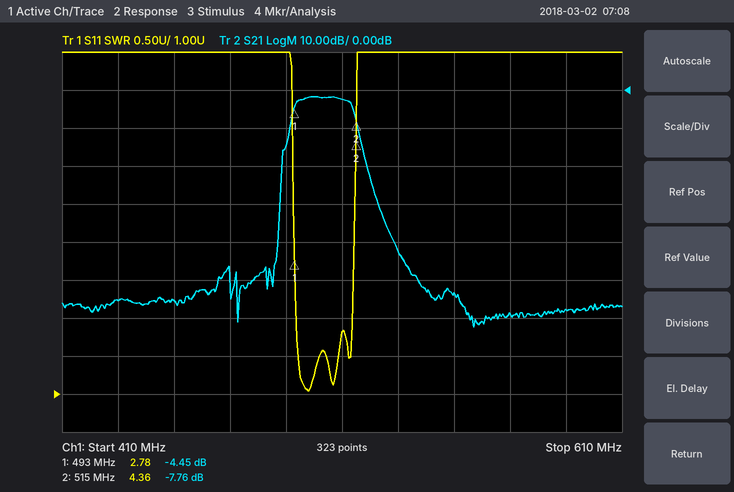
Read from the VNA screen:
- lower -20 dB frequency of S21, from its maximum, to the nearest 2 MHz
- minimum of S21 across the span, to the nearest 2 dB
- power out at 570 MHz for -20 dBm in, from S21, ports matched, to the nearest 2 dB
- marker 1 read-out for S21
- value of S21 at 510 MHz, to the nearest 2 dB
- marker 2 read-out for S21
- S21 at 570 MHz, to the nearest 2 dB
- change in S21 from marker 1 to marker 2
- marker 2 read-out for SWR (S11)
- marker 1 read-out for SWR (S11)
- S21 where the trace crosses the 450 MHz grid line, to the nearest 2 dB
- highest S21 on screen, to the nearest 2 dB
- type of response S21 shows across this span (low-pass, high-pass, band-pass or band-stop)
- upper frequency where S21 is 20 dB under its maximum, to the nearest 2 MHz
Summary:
488 MHz
-62 dB
-78 dBm
-4.45 dB
-2 dB
-7.76 dB
-58 dB
-3.31 dB
4.36
2.78
-56 dB
-2 dB
band-pass
520 MHz
